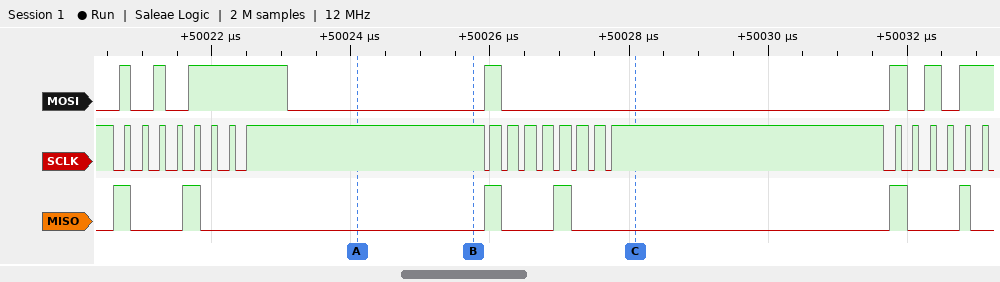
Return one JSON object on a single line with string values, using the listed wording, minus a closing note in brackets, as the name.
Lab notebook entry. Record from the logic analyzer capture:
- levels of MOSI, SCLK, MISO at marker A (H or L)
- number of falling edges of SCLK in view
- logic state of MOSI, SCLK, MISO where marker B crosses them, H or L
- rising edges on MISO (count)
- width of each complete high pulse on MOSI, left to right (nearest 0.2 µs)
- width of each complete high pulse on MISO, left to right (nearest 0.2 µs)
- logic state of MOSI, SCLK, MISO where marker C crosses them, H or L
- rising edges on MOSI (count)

{"levels of MOSI, SCLK, MISO at marker A": "MOSI=L, SCLK=H, MISO=L", "number of falling edges of SCLK in view": "23", "logic state of MOSI, SCLK, MISO where marker B crosses them, H or L": "MOSI=L, SCLK=H, MISO=L", "rising edges on MISO": "6", "width of each complete high pulse on MOSI, left to right": "0.2 µs, 0.2 µs, 1.4 µs, 0.2 µs, 0.2 µs, 0.2 µs", "width of each complete high pulse on MISO, left to right": "0.2 µs, 0.2 µs, 0.2 µs, 0.2 µs, 0.2 µs, 0.2 µs", "logic state of MOSI, SCLK, MISO where marker C crosses them, H or L": "MOSI=L, SCLK=H, MISO=L", "rising edges on MOSI": "7"}
